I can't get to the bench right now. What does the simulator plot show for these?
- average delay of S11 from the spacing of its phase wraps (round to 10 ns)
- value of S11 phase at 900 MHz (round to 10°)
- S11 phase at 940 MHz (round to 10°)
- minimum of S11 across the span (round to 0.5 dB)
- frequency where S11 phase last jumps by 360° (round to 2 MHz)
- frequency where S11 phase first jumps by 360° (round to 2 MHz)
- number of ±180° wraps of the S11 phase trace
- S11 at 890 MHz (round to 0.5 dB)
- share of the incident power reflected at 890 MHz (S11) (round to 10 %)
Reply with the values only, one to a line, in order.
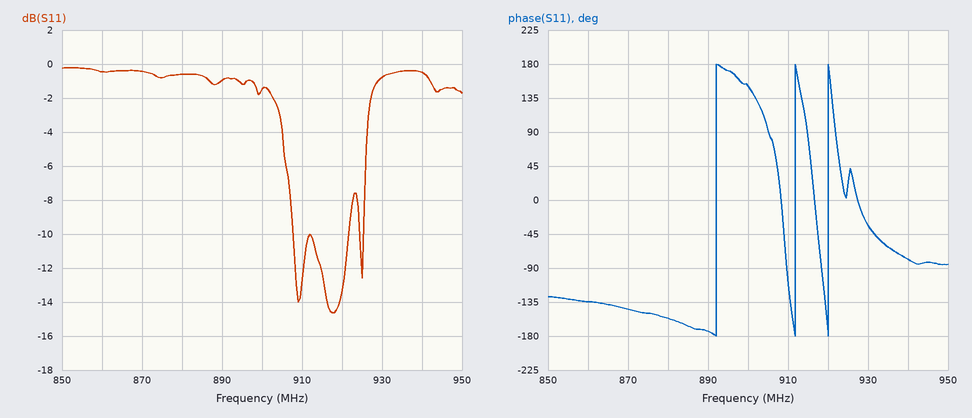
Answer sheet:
70 ns
150°
-80°
-14.5 dB
920 MHz
892 MHz
3
-1.0 dB
80 %
